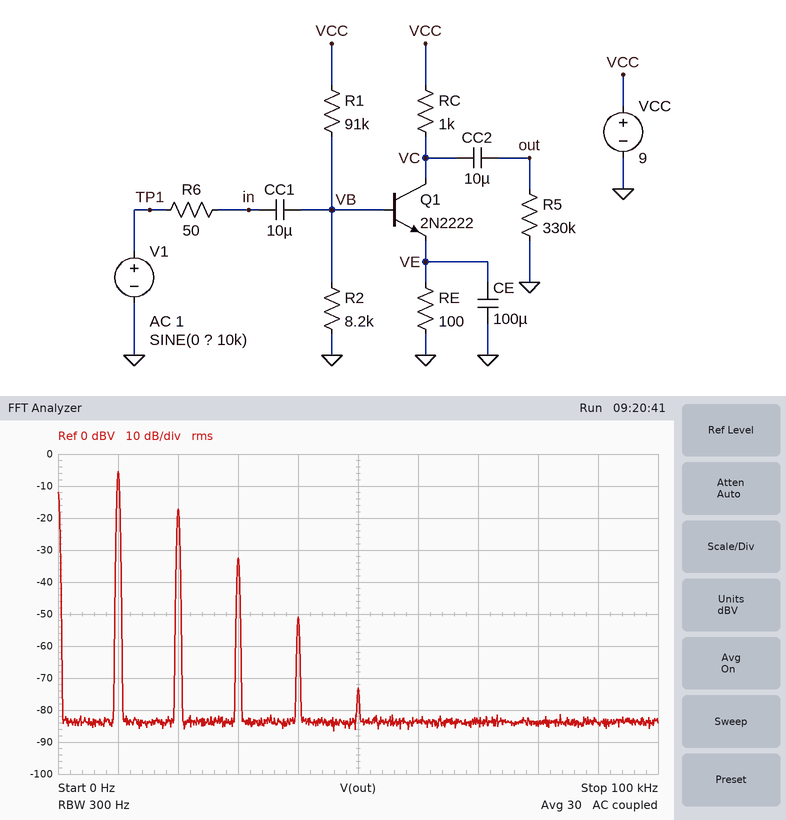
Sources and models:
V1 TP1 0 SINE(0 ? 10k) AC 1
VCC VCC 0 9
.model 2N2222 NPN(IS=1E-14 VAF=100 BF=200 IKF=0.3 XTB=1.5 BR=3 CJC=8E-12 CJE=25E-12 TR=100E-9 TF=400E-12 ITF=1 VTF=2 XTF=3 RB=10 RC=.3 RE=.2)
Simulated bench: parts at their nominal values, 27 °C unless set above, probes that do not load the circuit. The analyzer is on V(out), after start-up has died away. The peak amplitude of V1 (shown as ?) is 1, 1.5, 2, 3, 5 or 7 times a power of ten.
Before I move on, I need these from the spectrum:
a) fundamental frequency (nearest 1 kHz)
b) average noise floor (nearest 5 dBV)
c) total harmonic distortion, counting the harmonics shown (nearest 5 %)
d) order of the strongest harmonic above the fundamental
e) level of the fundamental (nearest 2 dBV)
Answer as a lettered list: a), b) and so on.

a) 10 kHz
b) -85 dBV
c) 25 %
d) 2
e) -6 dBV
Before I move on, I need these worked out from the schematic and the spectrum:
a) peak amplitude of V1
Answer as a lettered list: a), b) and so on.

a) 30 mV
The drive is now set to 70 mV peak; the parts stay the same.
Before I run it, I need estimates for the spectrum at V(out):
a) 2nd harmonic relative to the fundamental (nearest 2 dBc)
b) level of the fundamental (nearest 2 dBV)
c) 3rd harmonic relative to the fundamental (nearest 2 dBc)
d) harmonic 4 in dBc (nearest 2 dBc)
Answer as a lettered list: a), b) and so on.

a) -6 dBc
b) 0 dBV
c) -14 dBc
d) -26 dBc
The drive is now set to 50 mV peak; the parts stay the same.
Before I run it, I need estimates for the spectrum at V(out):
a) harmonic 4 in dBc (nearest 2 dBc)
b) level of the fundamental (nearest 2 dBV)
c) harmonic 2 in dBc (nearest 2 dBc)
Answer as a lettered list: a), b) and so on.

a) -34 dBc
b) -2 dBV
c) -8 dBc
